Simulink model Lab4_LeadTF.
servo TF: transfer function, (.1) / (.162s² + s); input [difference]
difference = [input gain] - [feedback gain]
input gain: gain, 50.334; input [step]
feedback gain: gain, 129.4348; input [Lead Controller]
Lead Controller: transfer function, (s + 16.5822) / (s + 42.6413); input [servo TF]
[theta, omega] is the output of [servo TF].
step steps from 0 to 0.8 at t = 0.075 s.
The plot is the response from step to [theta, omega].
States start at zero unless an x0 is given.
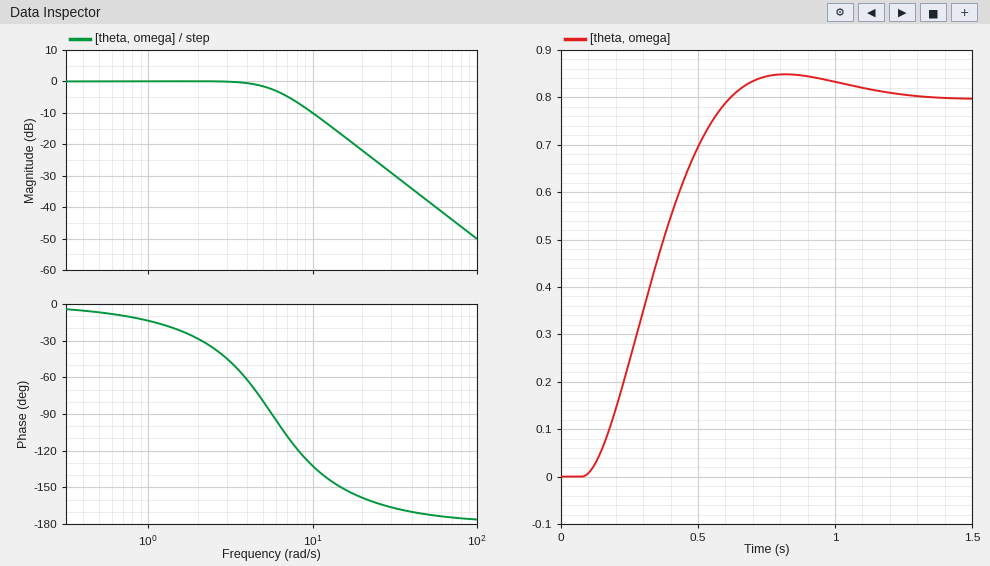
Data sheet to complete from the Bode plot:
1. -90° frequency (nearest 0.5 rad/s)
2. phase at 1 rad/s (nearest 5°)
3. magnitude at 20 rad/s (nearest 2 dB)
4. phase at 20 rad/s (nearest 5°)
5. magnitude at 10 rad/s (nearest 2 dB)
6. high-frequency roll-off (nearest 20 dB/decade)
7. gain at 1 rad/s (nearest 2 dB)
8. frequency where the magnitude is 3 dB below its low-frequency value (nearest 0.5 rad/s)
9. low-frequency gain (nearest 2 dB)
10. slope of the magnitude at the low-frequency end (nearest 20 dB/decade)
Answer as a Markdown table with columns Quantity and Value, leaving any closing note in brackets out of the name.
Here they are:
| Quantity | Value |
|---|---|
| -90° frequency | 5.5 rad/s |
| phase at 1 rad/s | -15° |
| magnitude at 20 rad/s | -22 dB |
| phase at 20 rad/s | -160° |
| magnitude at 10 rad/s | -10 dB |
| high-frequency roll-off | -40 dB/decade |
| gain at 1 rad/s | 0 dB |
| frequency where the magnitude is 3 dB below its low-frequency value | 6.0 rad/s |
| low-frequency gain | 0 dB |
| slope of the magnitude at the low-frequency end | 0 dB/decade |
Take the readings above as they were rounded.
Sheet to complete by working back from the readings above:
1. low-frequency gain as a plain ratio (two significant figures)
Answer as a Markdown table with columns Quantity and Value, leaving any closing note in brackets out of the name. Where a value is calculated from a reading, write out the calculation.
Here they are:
| Quantity | Value |
|---|---|
| low-frequency gain as a plain ratio | 10^(0 / 20) = 1.0 |
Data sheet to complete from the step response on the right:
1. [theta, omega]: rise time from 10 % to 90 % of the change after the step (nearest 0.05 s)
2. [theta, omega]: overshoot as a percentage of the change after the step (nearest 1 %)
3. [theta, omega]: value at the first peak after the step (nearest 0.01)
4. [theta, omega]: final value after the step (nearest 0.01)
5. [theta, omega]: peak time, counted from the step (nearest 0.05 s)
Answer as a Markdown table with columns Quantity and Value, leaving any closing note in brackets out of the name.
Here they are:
| Quantity | Value |
|---|---|
| [theta, omega]: rise time from 10 % to 90 % of the change after the step | 0.35 s |
| [theta, omega]: overshoot as a percentage of the change after the step | 6 % |
| [theta, omega]: value at the first peak after the step | 0.85 |
| [theta, omega]: final value after the step | 0.80 |
| [theta, omega]: peak time, counted from the step | 0.75 s |
